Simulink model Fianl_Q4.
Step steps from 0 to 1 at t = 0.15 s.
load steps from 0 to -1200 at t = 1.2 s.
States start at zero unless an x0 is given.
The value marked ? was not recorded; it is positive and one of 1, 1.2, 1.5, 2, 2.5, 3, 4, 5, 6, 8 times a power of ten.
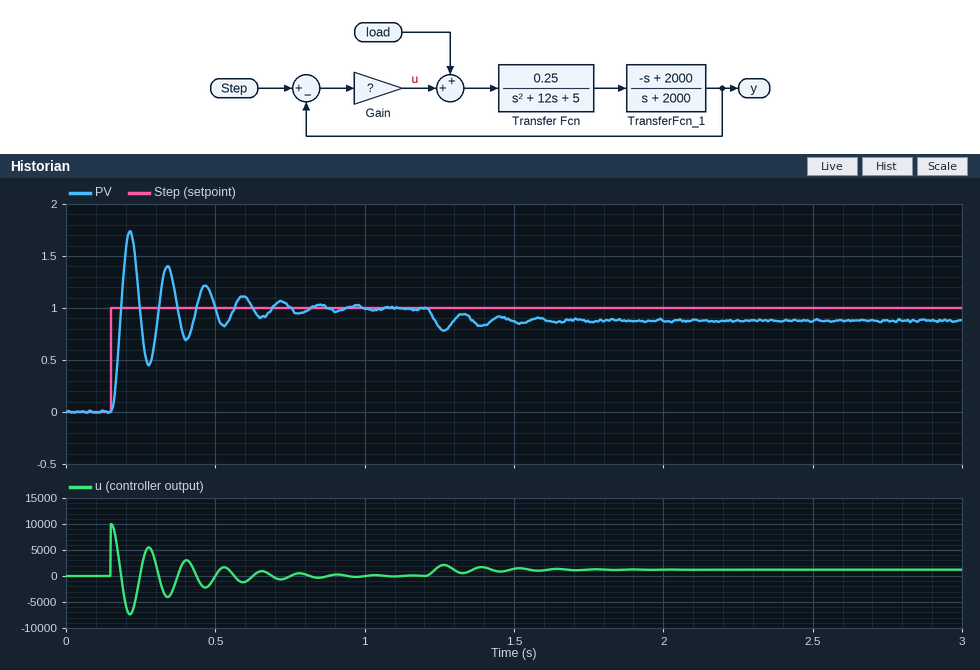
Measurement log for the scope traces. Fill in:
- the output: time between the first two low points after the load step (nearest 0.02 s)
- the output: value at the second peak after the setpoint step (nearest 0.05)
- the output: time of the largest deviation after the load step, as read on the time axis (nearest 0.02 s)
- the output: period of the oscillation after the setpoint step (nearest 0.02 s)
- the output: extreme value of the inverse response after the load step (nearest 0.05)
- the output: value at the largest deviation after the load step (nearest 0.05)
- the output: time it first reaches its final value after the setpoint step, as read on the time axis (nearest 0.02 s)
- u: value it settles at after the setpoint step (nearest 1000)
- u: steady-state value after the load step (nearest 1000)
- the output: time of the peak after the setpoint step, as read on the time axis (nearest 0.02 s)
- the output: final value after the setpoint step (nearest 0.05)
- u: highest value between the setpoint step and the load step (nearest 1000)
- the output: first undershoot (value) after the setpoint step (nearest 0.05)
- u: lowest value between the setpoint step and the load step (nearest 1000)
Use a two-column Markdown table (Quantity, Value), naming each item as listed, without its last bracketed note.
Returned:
| Quantity | Value |
|---|---|
| the output: time between the first two low points after the load step | 0.12 s |
| the output: value at the second peak after the setpoint step | 1.40 |
| the output: time of the largest deviation after the load step, as read on the time axis | 1.26 s |
| the output: period of the oscillation after the setpoint step | 0.12 s |
| the output: extreme value of the inverse response after the load step | 1.00 |
| the output: value at the largest deviation after the load step | 0.80 |
| the output: time it first reaches its final value after the setpoint step, as read on the time axis | 0.18 s |
| u: value it settles at after the setpoint step | 0 |
| u: steady-state value after the load step | 1000 |
| the output: time of the peak after the setpoint step, as read on the time axis | 0.22 s |
| the output: final value after the setpoint step | 1.00 |
| u: highest value between the setpoint step and the load step | 10000 |
| the output: first undershoot (value) after the setpoint step | 0.45 |
| u: lowest value between the setpoint step and the load step | -7000 |
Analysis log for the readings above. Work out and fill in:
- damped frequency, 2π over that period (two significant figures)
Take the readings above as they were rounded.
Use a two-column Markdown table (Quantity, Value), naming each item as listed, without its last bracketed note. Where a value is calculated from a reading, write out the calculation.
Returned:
| Quantity | Value |
|---|---|
| damped frequency, 2π over that period | 2π / 0.12 = 52 rad/s |
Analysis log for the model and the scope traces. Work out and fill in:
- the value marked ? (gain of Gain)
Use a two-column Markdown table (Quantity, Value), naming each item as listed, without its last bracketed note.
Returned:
| Quantity | Value |
|---|---|
| the value marked ? | 10000 |
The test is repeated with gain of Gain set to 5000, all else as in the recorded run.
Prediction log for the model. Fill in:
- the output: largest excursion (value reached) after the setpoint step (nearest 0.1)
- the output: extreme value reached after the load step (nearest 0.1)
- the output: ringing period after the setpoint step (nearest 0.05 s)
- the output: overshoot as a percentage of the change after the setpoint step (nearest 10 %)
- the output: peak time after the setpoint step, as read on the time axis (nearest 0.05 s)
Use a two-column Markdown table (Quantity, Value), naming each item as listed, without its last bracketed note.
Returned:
| Quantity | Value |
|---|---|
| the output: largest excursion (value reached) after the setpoint step | 1.6 |
| the output: extreme value reached after the load step | 0.6 |
| the output: ringing period after the setpoint step | 0.20 s |
| the output: overshoot as a percentage of the change after the setpoint step | 60 % |
| the output: peak time after the setpoint step, as read on the time axis | 0.25 s |
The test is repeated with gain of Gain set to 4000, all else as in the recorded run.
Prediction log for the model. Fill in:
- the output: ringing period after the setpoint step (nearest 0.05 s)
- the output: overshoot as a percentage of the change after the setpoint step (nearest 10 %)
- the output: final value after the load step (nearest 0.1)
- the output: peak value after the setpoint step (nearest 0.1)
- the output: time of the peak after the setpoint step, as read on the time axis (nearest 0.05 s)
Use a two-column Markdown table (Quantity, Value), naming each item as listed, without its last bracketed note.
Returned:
| Quantity | Value |
|---|---|
| the output: ringing period after the setpoint step | 0.20 s |
| the output: overshoot as a percentage of the change after the setpoint step | 60 % |
| the output: final value after the load step | 0.7 |
| the output: peak value after the setpoint step | 1.6 |
| the output: time of the peak after the setpoint step, as read on the time axis | 0.25 s |
